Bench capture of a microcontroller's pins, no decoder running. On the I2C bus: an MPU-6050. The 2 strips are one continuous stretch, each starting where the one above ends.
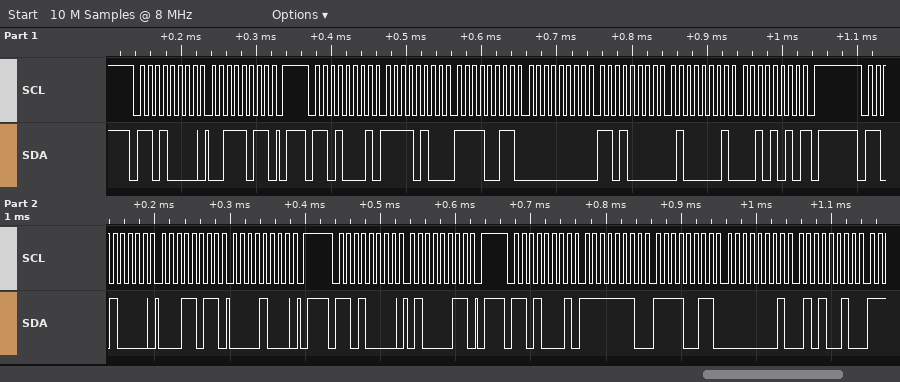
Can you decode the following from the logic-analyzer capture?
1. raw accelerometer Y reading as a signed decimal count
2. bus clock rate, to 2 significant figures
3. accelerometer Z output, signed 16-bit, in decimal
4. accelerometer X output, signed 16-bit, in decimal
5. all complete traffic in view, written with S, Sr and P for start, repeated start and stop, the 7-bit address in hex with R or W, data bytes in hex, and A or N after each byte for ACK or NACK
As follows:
208
100 kHz
16682
-2829
S 68W A 3B A P S 68R A F4 A F3 A 00 A D0 A 41 A 2A N P S 68W A 1B A 08 A P S 68W A 43 A P S 68R A FE A F3 A 01 A 52 A
